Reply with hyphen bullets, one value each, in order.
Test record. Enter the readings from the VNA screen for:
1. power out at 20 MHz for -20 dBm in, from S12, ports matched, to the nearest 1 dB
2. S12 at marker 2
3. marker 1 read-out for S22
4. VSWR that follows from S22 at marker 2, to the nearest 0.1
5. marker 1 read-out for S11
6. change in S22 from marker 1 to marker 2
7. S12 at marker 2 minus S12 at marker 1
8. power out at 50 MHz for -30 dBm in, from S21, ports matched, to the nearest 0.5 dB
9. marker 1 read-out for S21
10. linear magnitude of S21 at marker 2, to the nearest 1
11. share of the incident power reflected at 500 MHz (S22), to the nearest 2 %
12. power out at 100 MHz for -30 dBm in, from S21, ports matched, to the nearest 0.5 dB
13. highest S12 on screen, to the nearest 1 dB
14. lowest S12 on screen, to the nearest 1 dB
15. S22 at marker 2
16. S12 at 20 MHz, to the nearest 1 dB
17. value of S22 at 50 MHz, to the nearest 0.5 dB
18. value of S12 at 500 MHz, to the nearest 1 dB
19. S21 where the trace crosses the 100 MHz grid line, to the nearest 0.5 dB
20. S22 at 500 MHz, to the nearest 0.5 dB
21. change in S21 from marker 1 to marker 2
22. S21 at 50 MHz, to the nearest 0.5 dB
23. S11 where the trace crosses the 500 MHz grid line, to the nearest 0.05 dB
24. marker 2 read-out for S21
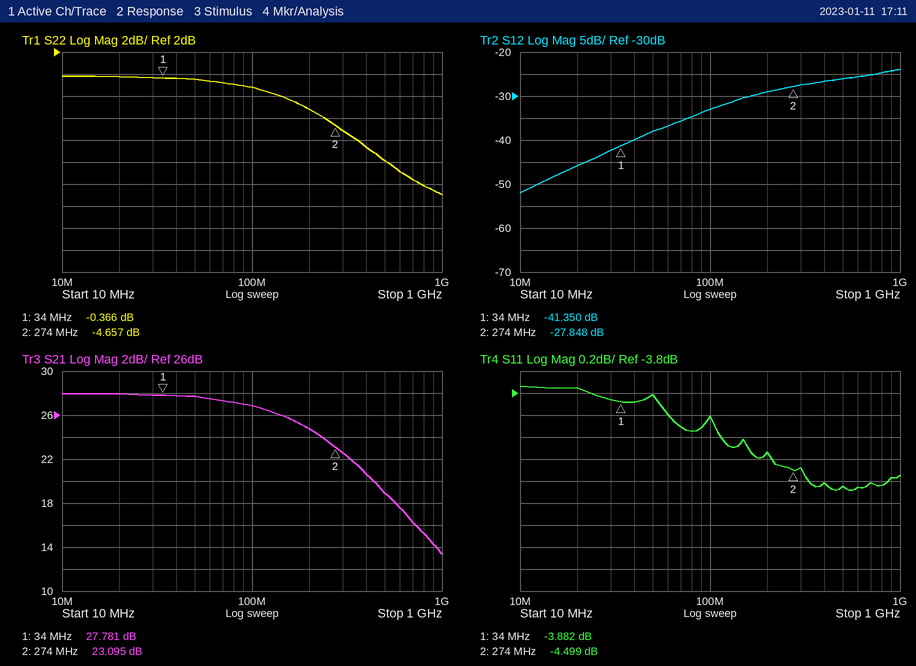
- -66 dBm
- -27.848 dB
- -0.366 dB
- 3.8
- -3.882 dB
- -4.291 dB
- 13.502 dB
- -2.5 dBm
- 27.781 dB
- 14
- 16 %
- -3.0 dBm
- -24 dB
- -52 dB
- -4.657 dB
- -46 dB
- -0.5 dB
- -26 dB
- 27.0 dB
- -8.0 dB
- -4.686 dB
- 27.5 dB
- -4.65 dB
- 23.095 dB
